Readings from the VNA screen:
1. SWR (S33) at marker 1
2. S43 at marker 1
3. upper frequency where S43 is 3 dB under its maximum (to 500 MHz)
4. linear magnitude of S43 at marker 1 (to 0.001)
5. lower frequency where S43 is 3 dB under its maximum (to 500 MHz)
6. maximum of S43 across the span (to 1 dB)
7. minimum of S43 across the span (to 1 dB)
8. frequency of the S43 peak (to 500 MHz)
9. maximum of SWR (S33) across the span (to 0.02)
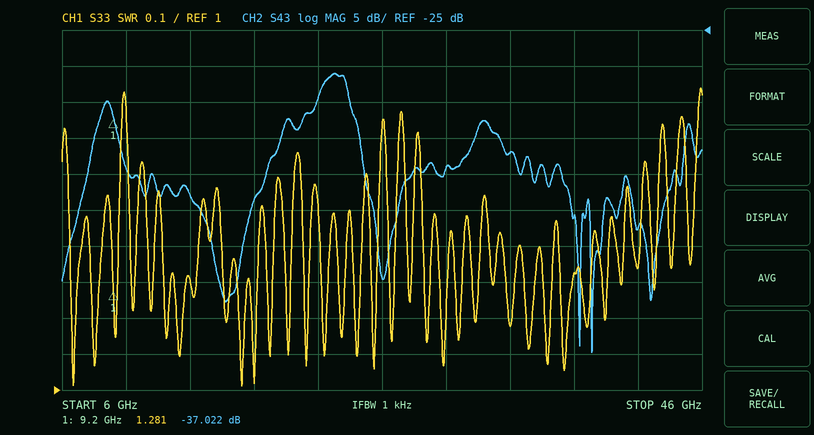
1.281
-37.022 dB
24.0 GHz
0.014
22.0 GHz
-31 dB
-70 dB
23.0 GHz
1.84
